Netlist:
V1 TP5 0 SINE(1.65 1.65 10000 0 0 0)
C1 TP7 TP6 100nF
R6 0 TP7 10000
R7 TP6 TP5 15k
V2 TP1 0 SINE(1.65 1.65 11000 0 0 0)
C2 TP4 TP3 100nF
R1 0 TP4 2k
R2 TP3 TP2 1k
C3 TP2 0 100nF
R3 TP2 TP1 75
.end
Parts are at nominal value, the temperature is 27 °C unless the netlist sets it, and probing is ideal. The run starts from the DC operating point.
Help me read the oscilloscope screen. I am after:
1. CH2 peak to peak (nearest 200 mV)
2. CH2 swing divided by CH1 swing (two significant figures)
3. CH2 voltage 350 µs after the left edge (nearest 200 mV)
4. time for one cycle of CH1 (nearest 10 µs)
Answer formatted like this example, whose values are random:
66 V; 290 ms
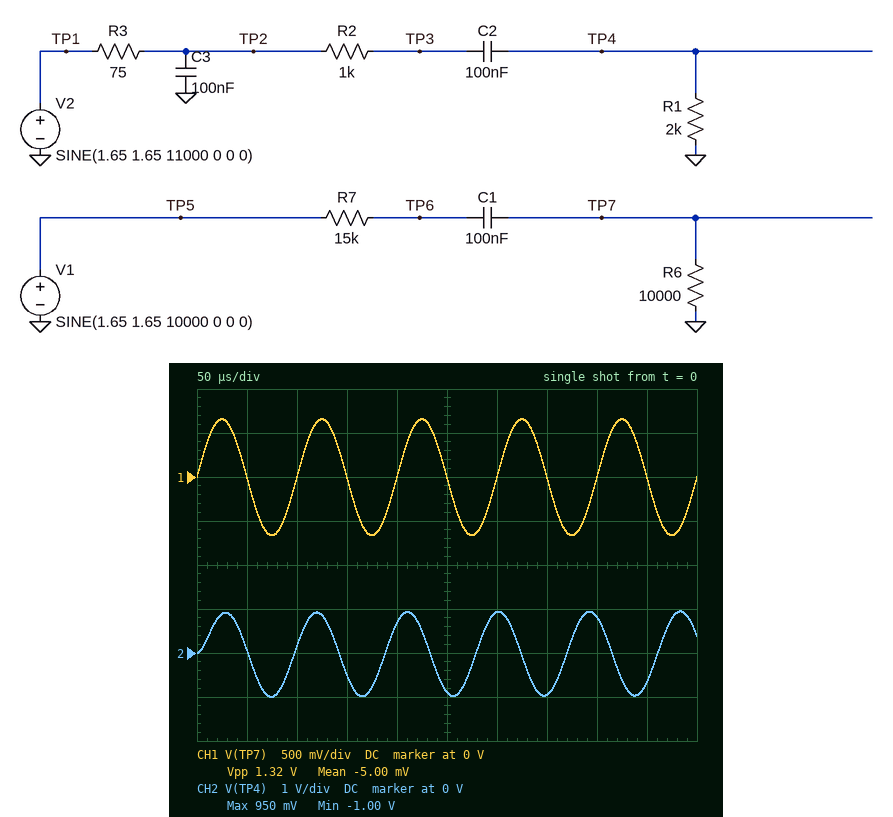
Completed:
2.0 V; 1.5; -1.0 V; 100 µs
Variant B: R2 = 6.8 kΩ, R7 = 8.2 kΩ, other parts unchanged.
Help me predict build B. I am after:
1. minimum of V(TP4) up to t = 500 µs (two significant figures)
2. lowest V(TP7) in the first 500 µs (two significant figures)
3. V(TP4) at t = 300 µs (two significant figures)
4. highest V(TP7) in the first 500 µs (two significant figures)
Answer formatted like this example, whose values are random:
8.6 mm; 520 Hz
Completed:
-340 mV; -910 mV; 320 mV; 900 mV
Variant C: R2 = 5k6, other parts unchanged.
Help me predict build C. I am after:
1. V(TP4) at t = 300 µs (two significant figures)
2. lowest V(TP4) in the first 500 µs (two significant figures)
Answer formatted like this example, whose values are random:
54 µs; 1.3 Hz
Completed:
370 mV; -390 mV
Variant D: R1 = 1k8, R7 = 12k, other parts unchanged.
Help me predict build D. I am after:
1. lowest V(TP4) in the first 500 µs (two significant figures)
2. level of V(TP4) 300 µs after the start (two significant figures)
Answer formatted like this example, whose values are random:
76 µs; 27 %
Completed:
-960 mV; 900 mV
